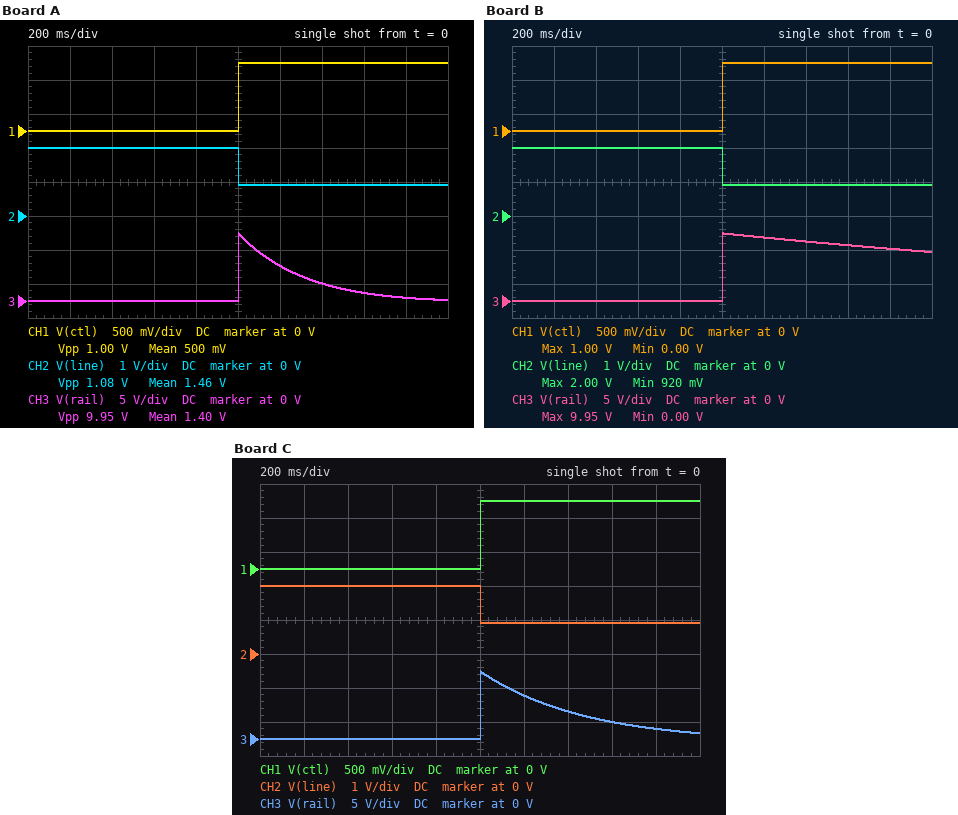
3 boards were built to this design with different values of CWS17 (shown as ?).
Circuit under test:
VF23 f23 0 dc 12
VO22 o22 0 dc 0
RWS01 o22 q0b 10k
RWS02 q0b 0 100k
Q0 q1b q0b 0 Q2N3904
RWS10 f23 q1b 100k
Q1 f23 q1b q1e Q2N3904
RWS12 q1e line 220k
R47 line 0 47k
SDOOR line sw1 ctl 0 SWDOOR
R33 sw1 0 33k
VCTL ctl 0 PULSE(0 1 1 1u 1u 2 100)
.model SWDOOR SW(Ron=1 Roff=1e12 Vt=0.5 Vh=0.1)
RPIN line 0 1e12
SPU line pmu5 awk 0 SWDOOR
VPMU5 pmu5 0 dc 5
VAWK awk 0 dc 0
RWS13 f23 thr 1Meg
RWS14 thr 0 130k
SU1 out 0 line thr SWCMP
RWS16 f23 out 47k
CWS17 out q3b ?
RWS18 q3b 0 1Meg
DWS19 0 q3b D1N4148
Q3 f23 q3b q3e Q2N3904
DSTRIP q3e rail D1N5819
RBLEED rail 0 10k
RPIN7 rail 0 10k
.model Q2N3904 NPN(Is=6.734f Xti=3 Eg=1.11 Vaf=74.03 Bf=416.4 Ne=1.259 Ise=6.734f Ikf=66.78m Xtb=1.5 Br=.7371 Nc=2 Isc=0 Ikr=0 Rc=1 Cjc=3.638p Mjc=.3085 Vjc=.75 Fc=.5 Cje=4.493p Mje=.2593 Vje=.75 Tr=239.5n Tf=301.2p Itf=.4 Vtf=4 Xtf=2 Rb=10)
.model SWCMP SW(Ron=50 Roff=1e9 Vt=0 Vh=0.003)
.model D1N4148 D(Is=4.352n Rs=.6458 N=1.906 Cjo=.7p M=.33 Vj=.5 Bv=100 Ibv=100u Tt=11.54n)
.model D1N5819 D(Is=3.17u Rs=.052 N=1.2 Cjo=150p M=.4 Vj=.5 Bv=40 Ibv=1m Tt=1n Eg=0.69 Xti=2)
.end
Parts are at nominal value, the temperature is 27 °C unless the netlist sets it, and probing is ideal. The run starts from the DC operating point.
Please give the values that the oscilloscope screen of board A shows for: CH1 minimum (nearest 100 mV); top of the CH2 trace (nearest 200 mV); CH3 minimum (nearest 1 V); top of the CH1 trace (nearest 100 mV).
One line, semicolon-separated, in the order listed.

0 V; 2.0 V; 0 V; 1.0 V
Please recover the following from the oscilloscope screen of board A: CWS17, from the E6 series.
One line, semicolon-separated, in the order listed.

680 nF
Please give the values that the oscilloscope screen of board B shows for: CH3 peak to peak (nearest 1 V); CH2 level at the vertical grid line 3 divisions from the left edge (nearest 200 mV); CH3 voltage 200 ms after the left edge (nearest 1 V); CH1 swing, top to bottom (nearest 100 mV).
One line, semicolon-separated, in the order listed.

10 V; 2.0 V; 0 V; 1.0 V
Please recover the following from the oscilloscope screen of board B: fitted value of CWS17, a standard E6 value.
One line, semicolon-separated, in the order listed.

6.8 µF
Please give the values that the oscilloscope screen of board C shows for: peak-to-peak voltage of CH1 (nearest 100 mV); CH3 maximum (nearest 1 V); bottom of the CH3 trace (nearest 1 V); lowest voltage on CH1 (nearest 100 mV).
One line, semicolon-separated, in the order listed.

1.0 V; 10 V; 0 V; 0 V
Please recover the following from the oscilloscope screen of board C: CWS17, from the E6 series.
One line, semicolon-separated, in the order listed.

1 µF
